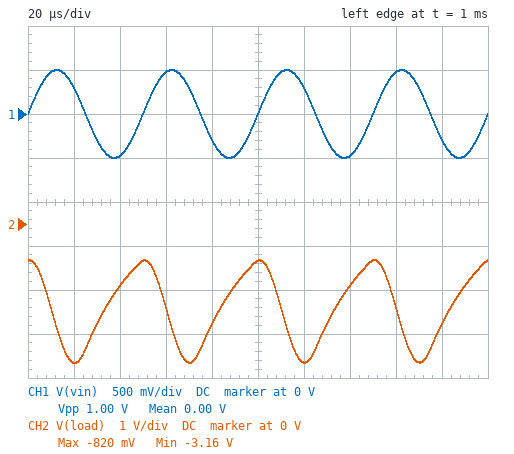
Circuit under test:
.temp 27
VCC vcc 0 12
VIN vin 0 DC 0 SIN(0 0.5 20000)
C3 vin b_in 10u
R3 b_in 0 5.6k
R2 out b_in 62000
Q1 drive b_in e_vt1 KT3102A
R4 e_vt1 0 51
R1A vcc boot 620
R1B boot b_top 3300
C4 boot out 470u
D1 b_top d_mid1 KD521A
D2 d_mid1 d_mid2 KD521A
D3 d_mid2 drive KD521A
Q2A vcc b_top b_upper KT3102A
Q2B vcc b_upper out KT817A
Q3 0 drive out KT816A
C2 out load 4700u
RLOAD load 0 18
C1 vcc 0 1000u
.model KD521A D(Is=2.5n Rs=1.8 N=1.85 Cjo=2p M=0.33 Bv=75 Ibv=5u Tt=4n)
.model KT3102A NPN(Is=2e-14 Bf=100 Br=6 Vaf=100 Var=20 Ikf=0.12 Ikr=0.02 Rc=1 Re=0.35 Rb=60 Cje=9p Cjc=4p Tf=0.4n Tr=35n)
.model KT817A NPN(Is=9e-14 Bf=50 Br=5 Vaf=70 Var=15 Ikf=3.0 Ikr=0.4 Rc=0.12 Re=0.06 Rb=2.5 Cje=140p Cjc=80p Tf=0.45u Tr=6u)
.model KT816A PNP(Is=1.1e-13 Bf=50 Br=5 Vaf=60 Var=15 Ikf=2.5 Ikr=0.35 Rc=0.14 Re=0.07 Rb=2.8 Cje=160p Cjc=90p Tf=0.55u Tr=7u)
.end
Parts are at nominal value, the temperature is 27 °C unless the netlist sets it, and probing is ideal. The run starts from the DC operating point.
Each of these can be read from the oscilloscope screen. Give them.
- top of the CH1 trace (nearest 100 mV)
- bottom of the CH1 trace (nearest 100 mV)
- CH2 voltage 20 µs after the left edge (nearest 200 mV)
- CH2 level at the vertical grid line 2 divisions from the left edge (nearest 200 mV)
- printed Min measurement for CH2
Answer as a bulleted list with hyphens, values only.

- 500 mV
- -500 mV
- -3.2 V
- -1.4 V
- -3.16 V
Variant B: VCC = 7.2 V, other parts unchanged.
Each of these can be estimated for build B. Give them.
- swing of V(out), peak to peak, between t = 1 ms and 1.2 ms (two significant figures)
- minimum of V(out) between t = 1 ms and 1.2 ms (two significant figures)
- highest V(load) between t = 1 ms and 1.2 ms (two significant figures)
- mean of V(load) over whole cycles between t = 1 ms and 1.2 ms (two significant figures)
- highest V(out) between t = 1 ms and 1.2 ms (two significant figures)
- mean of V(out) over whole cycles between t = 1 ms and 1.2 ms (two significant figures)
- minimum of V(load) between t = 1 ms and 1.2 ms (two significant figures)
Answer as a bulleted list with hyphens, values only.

- 1.5 V
- 3.9 V
- -680 mV
- -1.4 V
- 5.5 V
- 4.8 V
- -2.2 V
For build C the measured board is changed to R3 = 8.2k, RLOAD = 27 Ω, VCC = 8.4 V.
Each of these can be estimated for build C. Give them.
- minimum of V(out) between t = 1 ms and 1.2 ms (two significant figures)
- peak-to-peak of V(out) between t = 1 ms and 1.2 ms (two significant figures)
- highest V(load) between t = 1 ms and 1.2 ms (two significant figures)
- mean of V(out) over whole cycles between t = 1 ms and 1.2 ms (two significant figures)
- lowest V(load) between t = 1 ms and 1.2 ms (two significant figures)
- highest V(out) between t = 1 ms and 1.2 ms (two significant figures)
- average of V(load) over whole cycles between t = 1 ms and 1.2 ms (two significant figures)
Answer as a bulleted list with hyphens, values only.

- 1.3 V
- 3.2 V
- -1.2 V
- 3.0 V
- -4.4 V
- 4.5 V
- -2.7 V
